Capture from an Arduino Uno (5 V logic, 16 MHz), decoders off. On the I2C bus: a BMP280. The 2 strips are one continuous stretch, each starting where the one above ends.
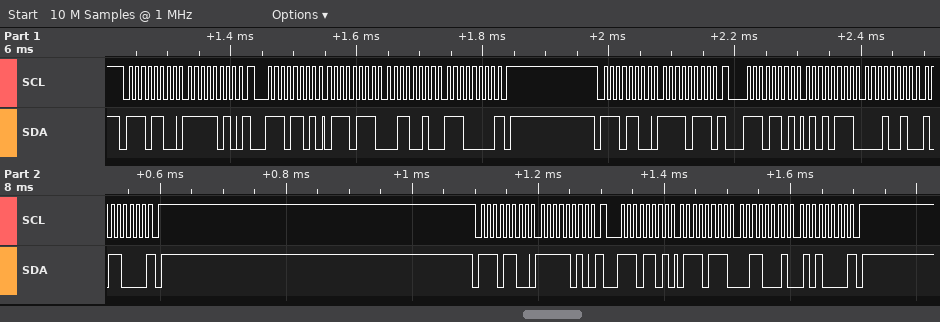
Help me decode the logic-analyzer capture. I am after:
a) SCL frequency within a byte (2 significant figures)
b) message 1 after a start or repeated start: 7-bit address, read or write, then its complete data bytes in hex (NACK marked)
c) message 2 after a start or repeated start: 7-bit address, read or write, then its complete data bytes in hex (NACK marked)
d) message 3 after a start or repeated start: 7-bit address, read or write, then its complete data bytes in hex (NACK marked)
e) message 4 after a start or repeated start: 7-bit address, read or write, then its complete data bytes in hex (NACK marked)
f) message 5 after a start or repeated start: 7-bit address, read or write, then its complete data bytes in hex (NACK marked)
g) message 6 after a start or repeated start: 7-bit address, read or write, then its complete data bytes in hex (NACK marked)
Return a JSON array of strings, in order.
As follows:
["100 kHz", "0x76 write: FA", "0x76 read: 77 32 E0 NACK", "0x76 write: F7", "0x76 read: 57 12 B0 NACK", "0x76 write: FA", "0x76 read: 77 31 50 NACK"]
